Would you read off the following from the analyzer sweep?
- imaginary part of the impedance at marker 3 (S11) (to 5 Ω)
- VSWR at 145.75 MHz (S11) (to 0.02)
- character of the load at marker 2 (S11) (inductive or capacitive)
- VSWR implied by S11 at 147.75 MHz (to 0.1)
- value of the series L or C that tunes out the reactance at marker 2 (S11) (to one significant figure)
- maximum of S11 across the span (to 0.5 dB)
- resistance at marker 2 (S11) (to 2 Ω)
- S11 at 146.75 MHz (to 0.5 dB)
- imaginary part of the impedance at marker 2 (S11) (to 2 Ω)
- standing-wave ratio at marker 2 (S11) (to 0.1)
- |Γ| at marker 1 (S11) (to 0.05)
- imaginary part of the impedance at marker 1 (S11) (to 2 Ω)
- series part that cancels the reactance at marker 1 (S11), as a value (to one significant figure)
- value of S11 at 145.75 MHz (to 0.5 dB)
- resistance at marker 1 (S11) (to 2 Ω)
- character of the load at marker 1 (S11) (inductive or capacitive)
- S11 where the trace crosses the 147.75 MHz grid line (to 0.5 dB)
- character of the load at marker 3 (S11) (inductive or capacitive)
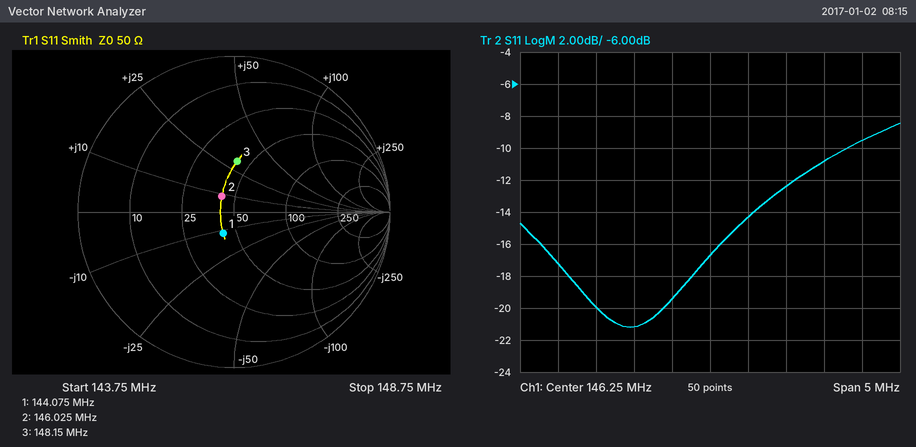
+30 Ω
1.24
inductive
1.8
100 pF
-8.5 dB
42 Ω
-14.5 dB
+8 Ω
1.3
0.15
-12 Ω
10 nH
-19.5 dB
42 Ω
capacitive
-11.0 dB
inductive
